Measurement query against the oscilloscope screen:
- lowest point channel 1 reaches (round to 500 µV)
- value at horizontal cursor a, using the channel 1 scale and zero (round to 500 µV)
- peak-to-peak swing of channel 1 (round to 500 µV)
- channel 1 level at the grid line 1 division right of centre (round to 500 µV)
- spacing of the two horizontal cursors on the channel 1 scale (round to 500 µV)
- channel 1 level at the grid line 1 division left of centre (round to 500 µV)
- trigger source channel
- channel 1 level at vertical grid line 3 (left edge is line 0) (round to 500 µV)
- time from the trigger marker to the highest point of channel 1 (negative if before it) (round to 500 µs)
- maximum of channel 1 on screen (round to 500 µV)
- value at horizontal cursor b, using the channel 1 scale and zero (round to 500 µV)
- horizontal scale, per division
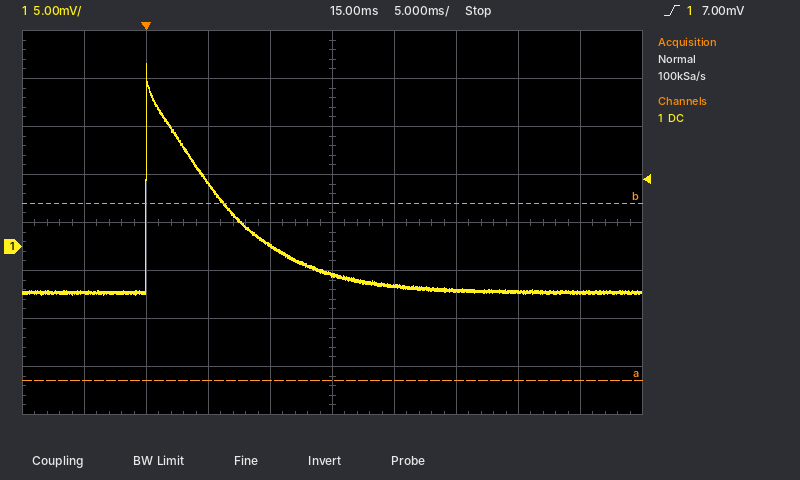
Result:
-5.0 mV
-14.0 mV
24.0 mV
-4.0 mV
18.5 mV
0.0 mV
channel 1
6.5 mV
0.0 ms
19.0 mV
4.5 mV
5 ms
